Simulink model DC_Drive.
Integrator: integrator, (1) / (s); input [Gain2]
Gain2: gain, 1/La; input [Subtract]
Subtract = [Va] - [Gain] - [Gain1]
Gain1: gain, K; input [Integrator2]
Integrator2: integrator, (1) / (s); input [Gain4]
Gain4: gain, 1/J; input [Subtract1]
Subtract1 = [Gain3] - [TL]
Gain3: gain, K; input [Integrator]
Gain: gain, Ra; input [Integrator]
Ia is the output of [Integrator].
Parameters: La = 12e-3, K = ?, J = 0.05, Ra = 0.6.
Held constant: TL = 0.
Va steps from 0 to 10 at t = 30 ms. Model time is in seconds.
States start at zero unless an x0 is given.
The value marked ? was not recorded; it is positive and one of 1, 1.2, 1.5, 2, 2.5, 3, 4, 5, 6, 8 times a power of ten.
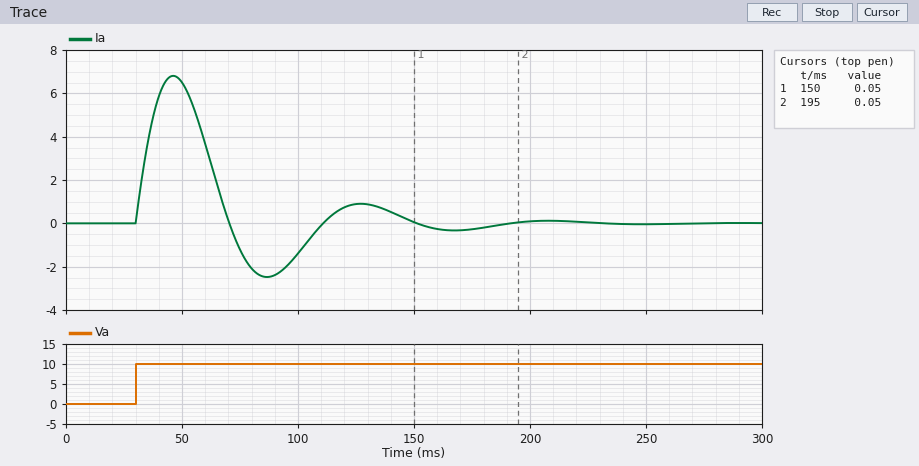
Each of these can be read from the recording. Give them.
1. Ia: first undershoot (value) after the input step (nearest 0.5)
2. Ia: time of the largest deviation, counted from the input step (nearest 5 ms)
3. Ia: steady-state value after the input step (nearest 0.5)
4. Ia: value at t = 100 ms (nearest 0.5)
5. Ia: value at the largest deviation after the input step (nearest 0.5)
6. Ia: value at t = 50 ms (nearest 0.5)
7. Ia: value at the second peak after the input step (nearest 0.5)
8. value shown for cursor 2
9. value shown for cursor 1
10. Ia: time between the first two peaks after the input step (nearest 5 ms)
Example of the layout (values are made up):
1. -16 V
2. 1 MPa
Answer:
1. -2.5
2. 15 ms
3. 0.0
4. -1.5
5. 7.0
6. 6.5
7. 1.0
8. 0.05
9. 0.05
10. 80 ms
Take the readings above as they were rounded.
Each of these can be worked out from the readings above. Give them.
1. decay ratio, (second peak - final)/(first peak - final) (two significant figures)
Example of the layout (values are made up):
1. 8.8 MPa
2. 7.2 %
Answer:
1. 0.14
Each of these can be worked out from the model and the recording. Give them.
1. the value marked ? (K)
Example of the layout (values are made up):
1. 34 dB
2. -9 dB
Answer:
1. 2
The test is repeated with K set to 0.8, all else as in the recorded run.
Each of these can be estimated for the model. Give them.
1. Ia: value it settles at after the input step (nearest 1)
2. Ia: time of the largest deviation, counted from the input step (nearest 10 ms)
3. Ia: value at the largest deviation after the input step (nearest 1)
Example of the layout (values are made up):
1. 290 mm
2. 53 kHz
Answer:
1. 0
2. 30 ms
3. 11
